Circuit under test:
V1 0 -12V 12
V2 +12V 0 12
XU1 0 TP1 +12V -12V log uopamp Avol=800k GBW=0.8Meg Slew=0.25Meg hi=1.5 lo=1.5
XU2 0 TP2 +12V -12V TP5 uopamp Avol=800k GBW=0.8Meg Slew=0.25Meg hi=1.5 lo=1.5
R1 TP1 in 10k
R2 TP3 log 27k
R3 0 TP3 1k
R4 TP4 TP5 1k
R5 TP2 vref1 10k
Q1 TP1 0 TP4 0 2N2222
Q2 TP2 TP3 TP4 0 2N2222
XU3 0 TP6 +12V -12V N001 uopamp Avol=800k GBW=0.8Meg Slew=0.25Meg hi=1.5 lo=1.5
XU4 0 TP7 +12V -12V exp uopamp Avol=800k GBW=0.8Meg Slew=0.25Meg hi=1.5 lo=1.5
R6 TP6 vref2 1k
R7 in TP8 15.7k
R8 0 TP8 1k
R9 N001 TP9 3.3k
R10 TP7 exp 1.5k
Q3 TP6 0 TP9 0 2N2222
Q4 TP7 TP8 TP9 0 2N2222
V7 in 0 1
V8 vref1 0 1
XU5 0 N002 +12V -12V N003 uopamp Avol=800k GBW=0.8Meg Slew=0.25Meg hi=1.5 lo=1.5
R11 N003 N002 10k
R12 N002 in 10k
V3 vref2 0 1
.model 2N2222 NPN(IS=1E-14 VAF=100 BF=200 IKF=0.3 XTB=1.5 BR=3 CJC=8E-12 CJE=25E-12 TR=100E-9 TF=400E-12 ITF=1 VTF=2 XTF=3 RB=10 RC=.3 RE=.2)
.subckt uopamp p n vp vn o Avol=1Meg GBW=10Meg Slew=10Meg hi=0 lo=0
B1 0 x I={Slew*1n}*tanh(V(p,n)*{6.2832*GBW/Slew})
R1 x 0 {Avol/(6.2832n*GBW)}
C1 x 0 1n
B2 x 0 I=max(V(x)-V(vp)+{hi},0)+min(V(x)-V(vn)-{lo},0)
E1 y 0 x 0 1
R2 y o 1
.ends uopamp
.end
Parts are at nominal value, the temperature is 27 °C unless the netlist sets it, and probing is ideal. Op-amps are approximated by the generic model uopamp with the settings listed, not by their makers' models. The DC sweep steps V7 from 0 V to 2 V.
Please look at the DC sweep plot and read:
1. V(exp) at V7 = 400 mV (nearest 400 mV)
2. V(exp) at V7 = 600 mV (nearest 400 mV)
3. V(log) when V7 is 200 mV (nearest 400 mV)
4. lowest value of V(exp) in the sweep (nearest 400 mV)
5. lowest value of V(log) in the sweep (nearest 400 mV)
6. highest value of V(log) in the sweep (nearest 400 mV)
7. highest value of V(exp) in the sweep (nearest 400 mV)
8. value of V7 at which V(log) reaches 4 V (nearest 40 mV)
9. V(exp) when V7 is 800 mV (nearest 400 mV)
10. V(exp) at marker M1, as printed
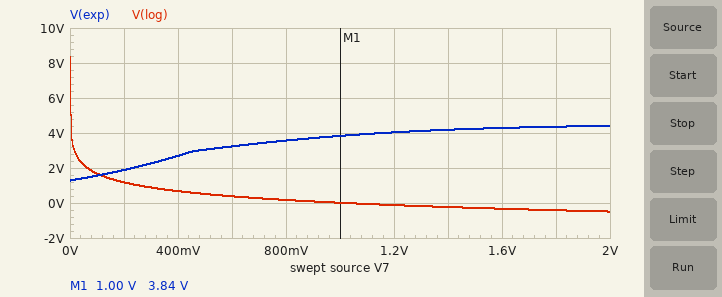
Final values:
2.8 V
3.2 V
1.2 V
1.2 V
-400 mV
8.4 V
4.4 V
0 V
3.6 V
3.84 V
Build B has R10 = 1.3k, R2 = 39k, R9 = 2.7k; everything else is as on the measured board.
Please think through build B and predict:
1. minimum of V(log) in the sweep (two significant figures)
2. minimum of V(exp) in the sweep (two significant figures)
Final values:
-700 mV
1.1 V
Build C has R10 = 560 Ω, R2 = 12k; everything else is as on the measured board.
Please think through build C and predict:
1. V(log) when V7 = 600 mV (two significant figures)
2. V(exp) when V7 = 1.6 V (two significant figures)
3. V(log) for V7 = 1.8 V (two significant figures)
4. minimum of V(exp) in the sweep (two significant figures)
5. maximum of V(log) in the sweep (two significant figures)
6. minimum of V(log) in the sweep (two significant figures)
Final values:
180 mV
1.6 V
-190 mV
480 mV
4.1 V
-230 mV
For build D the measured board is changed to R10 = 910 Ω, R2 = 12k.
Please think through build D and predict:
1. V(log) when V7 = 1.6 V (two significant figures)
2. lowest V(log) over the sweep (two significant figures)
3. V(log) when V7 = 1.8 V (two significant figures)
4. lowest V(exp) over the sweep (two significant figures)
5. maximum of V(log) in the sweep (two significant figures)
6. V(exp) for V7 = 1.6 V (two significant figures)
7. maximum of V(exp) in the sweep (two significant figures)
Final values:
-150 mV
-230 mV
-190 mV
780 mV
4.1 V
2.6 V
2.7 V
